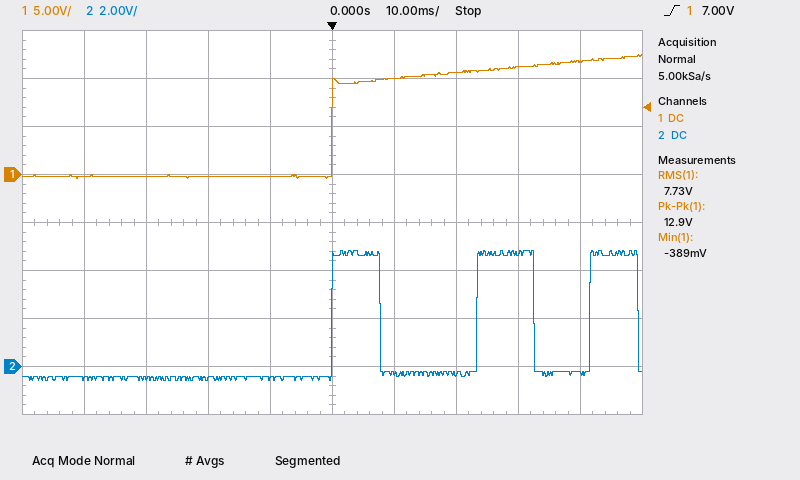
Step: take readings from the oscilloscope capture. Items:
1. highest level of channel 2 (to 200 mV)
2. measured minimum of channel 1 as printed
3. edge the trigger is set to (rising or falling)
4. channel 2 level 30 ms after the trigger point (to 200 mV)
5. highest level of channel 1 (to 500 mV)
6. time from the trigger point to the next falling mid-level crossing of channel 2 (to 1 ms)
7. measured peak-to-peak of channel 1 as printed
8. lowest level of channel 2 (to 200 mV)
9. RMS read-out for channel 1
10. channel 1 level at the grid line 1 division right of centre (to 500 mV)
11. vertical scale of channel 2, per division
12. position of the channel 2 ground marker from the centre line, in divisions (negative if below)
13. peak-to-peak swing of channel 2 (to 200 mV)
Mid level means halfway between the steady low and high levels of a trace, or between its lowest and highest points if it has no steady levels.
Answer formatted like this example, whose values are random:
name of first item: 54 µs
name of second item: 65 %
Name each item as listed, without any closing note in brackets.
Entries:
highest level of channel 2: 4.8 V
measured minimum of channel 1 as printed: -389 mV
edge the trigger is set to: rising
channel 2 level 30 ms after the trigger point: 4.8 V
highest level of channel 1: 12.5 V
time from the trigger point to the next falling mid-level crossing of channel 2: 8 ms
measured peak-to-peak of channel 1 as printed: 12.9 V
lowest level of channel 2: -600 mV
RMS read-out for channel 1: 7.73 V
channel 1 level at the grid line 1 division right of centre: 10.0 V
vertical scale of channel 2, per division: 2 V
position of the channel 2 ground marker from the centre line, in divisions: -3.0 div
peak-to-peak swing of channel 2: 5.4 V
